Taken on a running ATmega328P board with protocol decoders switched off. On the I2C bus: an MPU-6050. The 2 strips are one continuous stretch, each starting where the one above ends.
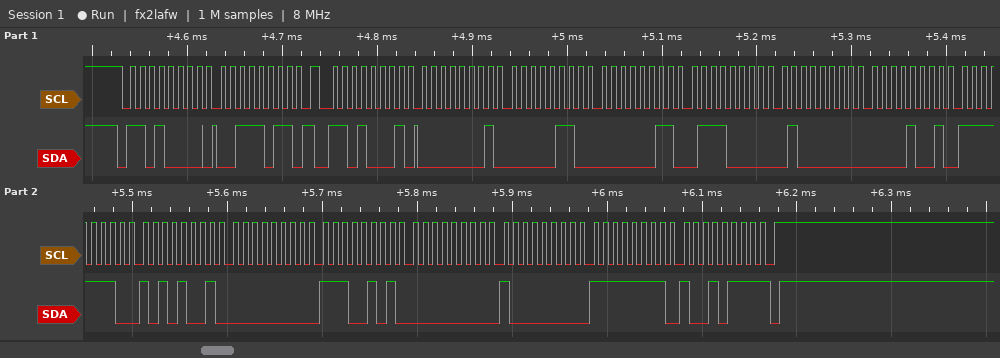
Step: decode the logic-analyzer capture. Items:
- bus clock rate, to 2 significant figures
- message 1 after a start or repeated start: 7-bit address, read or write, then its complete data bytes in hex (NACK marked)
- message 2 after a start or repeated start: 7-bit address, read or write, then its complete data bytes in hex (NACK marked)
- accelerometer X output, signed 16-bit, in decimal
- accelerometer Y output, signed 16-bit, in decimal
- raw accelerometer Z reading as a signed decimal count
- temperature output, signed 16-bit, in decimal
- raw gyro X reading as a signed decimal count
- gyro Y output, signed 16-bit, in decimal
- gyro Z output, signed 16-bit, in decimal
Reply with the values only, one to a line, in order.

100 kHz
0x68 write: 3B
0x68 read: 01 06 03 70 40 09 FE A9 00 E5 00 80 FF 97 NACK
262
880
16393
-343
229
128
-105
